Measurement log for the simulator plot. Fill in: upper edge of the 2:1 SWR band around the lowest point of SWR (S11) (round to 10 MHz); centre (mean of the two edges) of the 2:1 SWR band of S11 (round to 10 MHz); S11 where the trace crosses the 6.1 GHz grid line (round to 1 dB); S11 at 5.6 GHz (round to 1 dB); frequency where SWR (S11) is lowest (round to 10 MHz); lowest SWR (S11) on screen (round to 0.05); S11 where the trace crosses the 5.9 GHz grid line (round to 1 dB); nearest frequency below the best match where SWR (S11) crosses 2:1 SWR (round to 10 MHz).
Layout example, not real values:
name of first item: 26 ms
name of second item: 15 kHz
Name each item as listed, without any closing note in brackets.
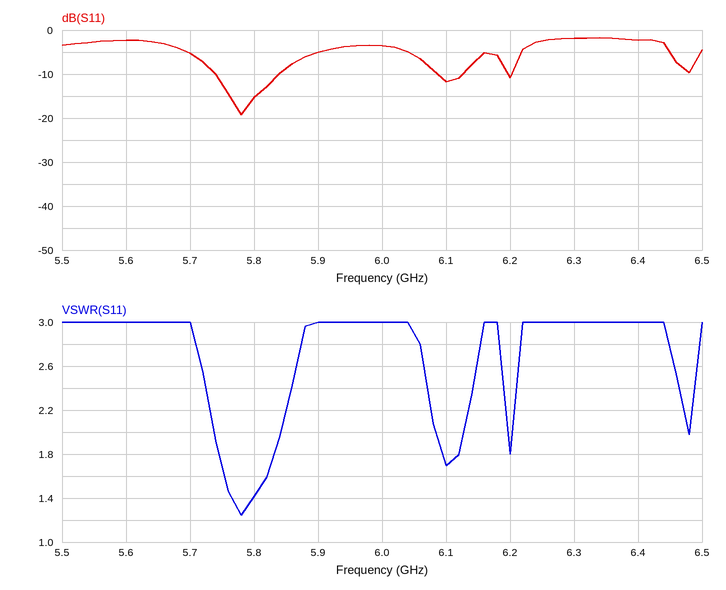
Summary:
upper edge of the 2:1 SWR band around the lowest point of SWR (S11): 5.84 GHz
centre (mean of the two edges) of the 2:1 SWR band of S11: 5.79 GHz
S11 where the trace crosses the 6.1 GHz grid line: -12 dB
S11 at 5.6 GHz: -2 dB
frequency where SWR (S11) is lowest: 5.78 GHz
lowest SWR (S11) on screen: 1.25
S11 where the trace crosses the 5.9 GHz grid line: -5 dB
nearest frequency below the best match where SWR (S11) crosses 2:1 SWR: 5.74 GHz
